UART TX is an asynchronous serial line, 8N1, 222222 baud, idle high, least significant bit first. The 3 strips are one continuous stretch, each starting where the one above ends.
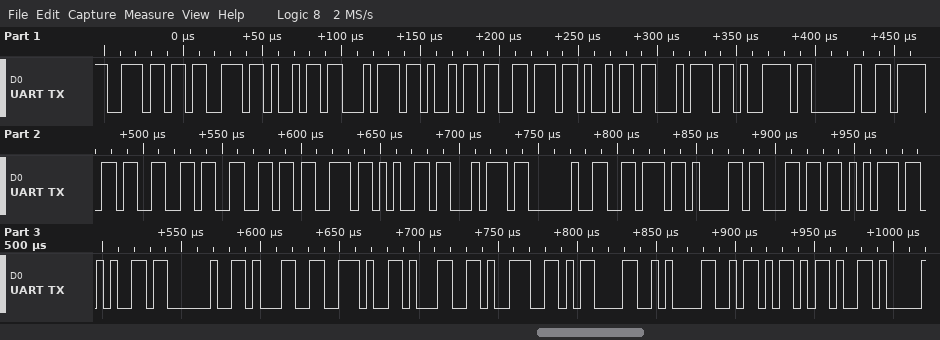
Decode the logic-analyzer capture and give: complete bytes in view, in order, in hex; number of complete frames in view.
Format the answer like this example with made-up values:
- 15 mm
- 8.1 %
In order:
- 6E 73 69 74 69 76 69 74 79 20 6F 66 66 73 65 74 20 76 61 6C 75 65 20 31 2E 31 39 0D 0A 5A 2D
- 31
